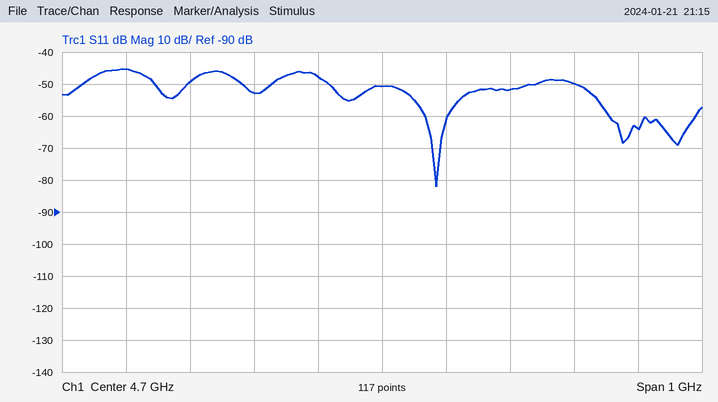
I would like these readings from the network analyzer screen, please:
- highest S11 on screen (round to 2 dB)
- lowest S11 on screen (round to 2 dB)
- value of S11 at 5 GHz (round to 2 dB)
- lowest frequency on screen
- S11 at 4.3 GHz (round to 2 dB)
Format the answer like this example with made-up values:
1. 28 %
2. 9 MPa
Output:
1. -46 dB
2. -82 dB
3. -50 dB
4. 4.2 GHz
5. -46 dB
